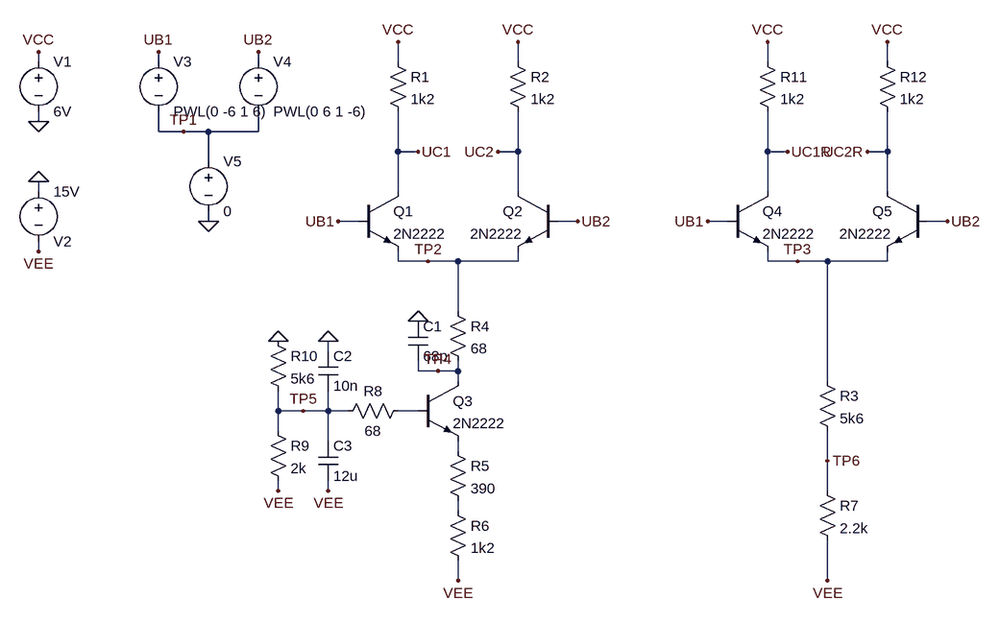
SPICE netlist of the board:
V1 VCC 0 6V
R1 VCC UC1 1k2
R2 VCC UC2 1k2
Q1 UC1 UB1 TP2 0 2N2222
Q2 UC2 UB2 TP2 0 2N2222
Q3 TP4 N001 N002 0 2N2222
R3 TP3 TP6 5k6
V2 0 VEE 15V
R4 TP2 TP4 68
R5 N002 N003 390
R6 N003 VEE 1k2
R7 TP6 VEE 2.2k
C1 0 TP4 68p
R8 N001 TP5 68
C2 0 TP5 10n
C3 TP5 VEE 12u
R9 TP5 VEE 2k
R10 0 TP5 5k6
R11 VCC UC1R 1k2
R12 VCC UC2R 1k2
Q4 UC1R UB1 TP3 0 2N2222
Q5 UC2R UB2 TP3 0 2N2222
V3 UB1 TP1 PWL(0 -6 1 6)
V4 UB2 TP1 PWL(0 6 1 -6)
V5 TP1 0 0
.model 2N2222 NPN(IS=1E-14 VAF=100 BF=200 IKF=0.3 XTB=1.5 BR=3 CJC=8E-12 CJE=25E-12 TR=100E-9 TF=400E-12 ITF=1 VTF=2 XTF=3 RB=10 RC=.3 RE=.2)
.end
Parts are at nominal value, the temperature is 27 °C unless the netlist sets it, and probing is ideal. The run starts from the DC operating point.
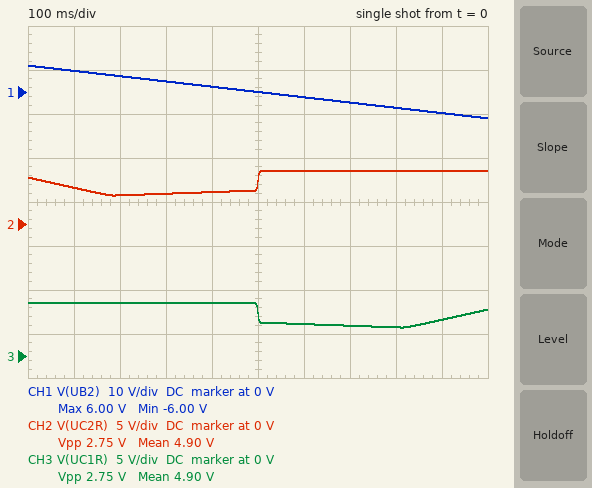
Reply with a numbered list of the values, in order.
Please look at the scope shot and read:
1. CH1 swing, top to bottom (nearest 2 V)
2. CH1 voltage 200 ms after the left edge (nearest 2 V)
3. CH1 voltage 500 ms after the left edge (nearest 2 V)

1. 12 V
2. 4 V
3. 0 V
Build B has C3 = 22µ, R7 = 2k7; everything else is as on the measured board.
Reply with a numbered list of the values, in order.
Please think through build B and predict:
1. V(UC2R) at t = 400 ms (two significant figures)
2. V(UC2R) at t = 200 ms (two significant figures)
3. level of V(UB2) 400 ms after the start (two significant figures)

1. 3.8 V
2. 3.4 V
3. 1.2 V
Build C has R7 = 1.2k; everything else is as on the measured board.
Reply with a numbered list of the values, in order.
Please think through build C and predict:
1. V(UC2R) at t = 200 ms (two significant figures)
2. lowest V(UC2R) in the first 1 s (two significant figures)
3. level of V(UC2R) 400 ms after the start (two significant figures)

1. 3.0 V
2. 2.9 V
3. 3.3 V
